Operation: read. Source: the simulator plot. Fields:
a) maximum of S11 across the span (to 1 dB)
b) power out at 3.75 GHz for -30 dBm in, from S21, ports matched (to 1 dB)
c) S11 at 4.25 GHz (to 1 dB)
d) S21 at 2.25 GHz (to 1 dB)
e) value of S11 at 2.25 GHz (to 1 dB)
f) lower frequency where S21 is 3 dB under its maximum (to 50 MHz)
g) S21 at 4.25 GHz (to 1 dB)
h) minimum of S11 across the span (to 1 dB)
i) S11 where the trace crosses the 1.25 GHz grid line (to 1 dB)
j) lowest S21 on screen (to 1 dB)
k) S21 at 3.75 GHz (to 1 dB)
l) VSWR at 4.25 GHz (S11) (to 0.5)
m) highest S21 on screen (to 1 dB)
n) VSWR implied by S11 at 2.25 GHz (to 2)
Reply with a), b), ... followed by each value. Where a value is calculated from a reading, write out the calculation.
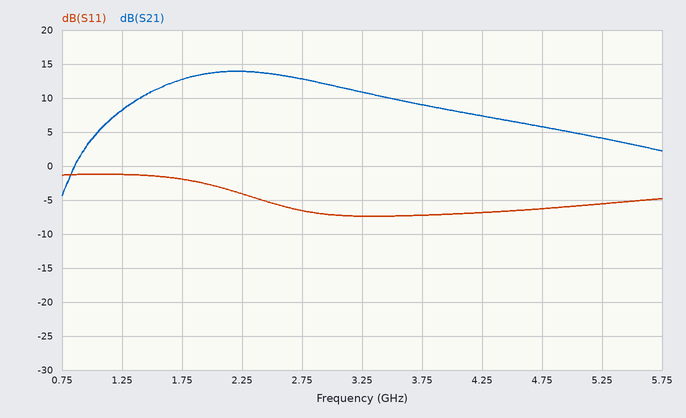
a) -1 dB
b) -30 dBm + (9 dB) = -21 dBm
c) -7 dB
d) 14 dB
e) -4 dB
f) 1.50 GHz
g) 7 dB
h) -7 dB
i) -1 dB
j) -4 dB
k) 9 dB
l) |Γ| = 10^(-7/20) = 0.4467; VSWR = (1 + 0.4467)/(1 − 0.4467) ≈ 2.61, so 2.5 to the nearest 0.5
m) 14 dB
n) |Γ| = 10^(-4/20) = 0.6310; VSWR = (1 + 0.6310)/(1 − 0.6310) ≈ 4
